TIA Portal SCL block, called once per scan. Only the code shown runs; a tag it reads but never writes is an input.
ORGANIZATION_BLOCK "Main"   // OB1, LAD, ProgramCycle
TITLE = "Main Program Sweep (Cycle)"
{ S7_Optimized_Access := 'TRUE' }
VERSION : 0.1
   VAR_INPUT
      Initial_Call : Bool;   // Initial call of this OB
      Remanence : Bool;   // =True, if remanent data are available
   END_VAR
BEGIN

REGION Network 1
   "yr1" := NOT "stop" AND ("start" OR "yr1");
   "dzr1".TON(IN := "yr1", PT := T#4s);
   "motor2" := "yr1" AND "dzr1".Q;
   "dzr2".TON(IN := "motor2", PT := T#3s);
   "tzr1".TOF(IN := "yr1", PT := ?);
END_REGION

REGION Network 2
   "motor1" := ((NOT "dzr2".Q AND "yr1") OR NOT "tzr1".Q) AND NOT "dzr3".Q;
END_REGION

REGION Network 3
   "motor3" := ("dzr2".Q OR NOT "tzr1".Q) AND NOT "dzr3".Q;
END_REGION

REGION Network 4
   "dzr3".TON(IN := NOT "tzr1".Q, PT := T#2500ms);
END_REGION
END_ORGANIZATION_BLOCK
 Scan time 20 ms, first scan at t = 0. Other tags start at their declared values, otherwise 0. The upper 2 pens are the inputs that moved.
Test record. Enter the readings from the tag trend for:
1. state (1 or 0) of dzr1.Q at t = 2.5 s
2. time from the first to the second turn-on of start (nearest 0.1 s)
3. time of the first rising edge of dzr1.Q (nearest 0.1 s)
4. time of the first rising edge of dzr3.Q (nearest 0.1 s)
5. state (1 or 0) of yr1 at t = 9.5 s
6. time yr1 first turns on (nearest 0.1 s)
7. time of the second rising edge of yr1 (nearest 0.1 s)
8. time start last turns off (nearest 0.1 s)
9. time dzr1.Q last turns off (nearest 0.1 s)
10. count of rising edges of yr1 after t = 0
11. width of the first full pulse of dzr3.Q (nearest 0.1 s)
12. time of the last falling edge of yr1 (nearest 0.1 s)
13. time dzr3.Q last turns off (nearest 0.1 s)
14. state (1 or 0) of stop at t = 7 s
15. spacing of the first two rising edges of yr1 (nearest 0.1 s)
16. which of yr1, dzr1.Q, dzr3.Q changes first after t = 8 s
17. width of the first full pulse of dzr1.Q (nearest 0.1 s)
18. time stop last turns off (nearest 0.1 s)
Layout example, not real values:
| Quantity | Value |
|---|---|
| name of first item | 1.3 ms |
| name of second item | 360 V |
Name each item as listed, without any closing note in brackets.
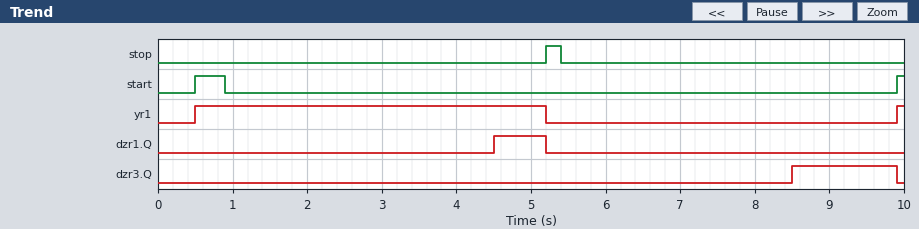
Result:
| Quantity | Value |
|---|---|
| state (1 or 0) of dzr1.Q at t = 2.5 s | 0 |
| time from the first to the second turn-on of start | 9.4 s |
| time of the first rising edge of dzr1.Q | 4.5 s |
| time of the first rising edge of dzr3.Q | 8.5 s |
| state (1 or 0) of yr1 at t = 9.5 s | 0 |
| time yr1 first turns on | 0.5 s |
| time of the second rising edge of yr1 | 9.9 s |
| time start last turns off | 0.9 s |
| time dzr1.Q last turns off | 5.2 s |
| count of rising edges of yr1 after t = 0 | 2 |
| width of the first full pulse of dzr3.Q | 1.4 s |
| time of the last falling edge of yr1 | 5.2 s |
| time dzr3.Q last turns off | 9.9 s |
| state (1 or 0) of stop at t = 7 s | 0 |
| spacing of the first two rising edges of yr1 | 9.4 s |
| which of yr1, dzr1.Q, dzr3.Q changes first after t = 8 s | dzr3.Q |
| width of the first full pulse of dzr1.Q | 0.7 s |
| time stop last turns off | 5.4 s |
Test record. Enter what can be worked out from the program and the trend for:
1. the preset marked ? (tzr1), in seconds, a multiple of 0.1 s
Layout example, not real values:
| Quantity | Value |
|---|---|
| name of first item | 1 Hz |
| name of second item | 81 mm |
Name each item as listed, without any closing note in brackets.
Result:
| Quantity | Value |
|---|---|
| the preset marked ? (tzr1), in seconds, a multiple of 0.1 s | 0.8 s |
